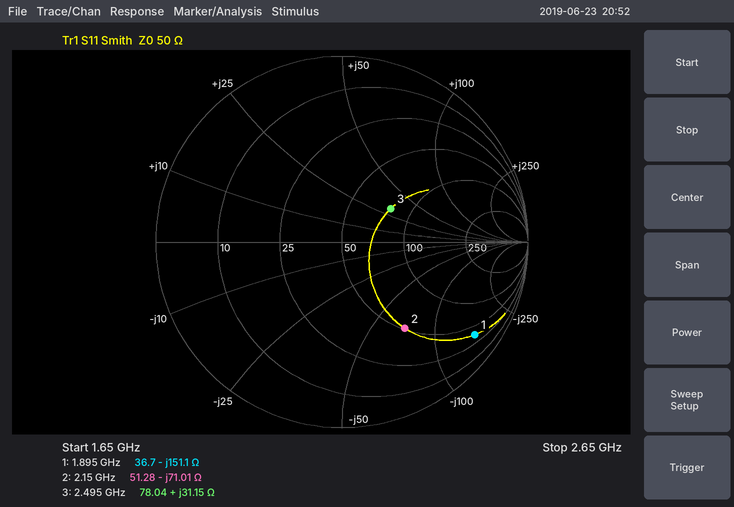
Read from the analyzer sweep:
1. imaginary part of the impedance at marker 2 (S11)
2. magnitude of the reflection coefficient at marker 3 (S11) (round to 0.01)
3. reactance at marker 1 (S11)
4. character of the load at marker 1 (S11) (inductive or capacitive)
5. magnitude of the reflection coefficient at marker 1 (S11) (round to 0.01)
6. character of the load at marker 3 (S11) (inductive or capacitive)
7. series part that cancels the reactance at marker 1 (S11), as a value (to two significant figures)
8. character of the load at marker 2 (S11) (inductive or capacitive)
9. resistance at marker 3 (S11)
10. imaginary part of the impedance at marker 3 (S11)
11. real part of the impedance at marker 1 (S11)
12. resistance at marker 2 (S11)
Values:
-71.01 Ω
0.32
-151.1 Ω
capacitive
0.87
inductive
13 nH
capacitive
78.04 Ω
+31.15 Ω
36.7 Ω
51.28 Ω
